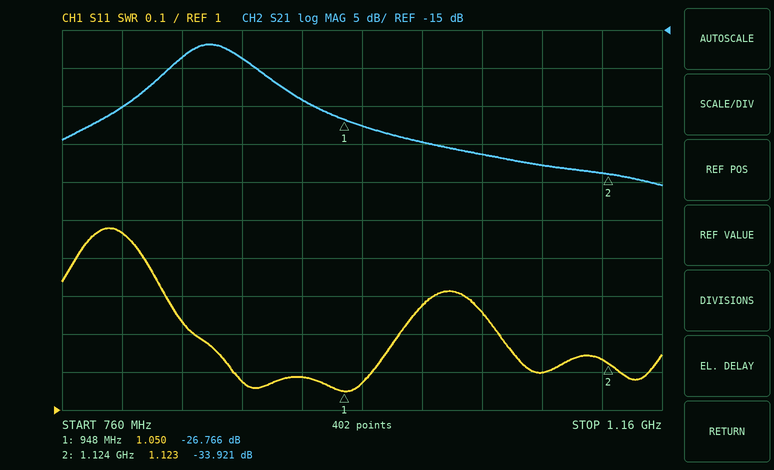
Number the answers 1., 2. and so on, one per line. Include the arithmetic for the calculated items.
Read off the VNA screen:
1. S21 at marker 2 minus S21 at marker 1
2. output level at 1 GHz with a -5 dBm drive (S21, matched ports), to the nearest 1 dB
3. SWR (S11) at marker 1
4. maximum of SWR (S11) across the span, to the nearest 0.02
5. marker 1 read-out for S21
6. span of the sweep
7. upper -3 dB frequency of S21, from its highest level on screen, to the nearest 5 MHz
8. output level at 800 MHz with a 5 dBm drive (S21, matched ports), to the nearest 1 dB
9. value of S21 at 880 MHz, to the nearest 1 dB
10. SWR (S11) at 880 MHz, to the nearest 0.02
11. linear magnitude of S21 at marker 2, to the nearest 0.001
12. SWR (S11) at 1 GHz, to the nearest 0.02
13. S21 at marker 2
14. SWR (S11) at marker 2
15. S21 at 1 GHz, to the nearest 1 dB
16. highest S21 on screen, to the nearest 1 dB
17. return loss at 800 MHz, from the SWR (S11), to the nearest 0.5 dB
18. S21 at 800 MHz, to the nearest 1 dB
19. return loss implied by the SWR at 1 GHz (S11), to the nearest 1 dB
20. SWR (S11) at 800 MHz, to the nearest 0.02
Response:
1. -33.921 − (-26.766) = -7.155 dB
2. -5 dBm + (-30 dB) = -35 dBm
3. 1.050
4. 1.48
5. -26.766 dB
6. 400 MHz
7. 890 MHz
8. 5 dBm + (-25 dB) = -20 dBm
9. -19 dB
10. 1.08
11. 10^(-33.921/20) ≈ 0.020
12. 1.28
13. -33.921 dB
14. 1.123
15. -30 dB
16. -17 dB
17. −20 log10((1.46 − 1)/(1.46 + 1)) ≈ 14.6 dB, so 14.5 dB to the nearest 0.5 dB
18. -25 dB
19. −20 log10((1.28 − 1)/(1.28 + 1)) ≈ 18 dB
20. 1.46
